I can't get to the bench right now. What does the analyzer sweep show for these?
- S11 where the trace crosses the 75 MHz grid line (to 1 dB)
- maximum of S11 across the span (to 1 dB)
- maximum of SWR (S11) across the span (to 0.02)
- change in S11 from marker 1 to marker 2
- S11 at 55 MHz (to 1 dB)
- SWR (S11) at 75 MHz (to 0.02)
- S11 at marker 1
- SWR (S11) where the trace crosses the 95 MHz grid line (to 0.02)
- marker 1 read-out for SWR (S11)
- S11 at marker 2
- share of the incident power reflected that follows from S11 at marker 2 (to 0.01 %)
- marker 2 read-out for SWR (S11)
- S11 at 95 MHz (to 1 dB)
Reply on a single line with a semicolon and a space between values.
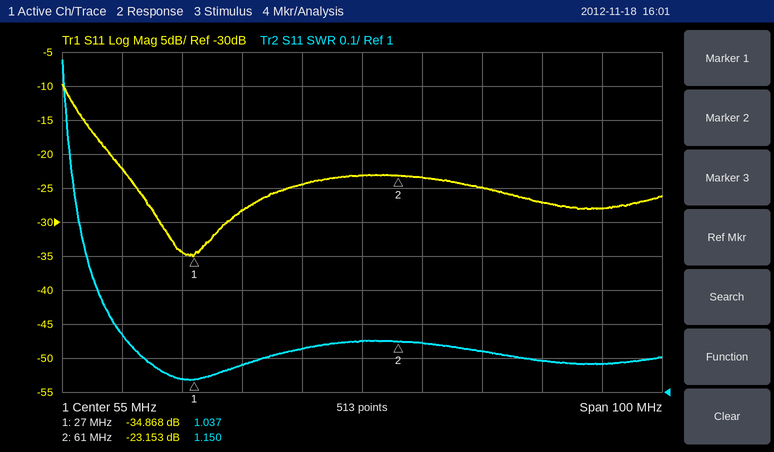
-25 dB; -10 dB; 1.98; 11.715 dB; -23 dB; 1.12; -34.868 dB; 1.08; 1.037; -23.153 dB; 0.48 %; 1.150; -28 dB
